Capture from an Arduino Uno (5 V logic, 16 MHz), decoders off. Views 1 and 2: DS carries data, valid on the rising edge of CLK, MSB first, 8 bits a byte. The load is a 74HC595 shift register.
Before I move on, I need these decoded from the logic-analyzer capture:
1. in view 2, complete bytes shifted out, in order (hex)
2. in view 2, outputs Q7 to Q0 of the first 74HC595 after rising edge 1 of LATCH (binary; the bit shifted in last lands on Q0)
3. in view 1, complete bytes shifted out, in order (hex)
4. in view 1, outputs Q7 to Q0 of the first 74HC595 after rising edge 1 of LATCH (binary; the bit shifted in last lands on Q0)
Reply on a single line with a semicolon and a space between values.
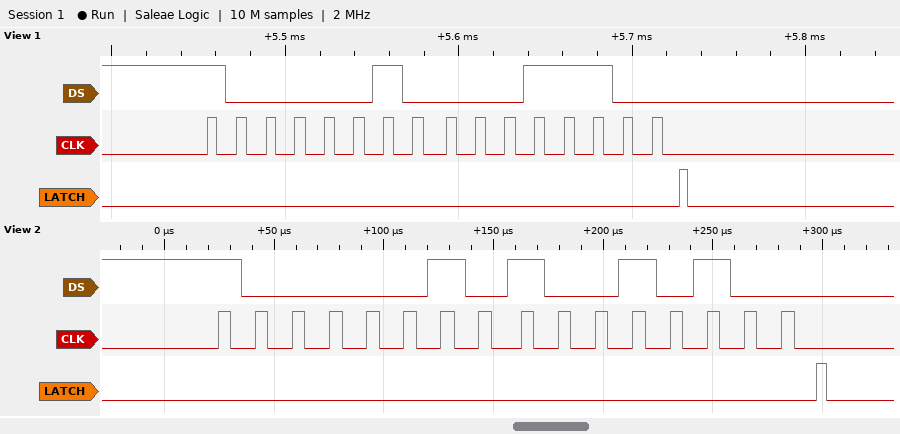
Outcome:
82 94; 10010100; 0x82 0x1C; 00011100
